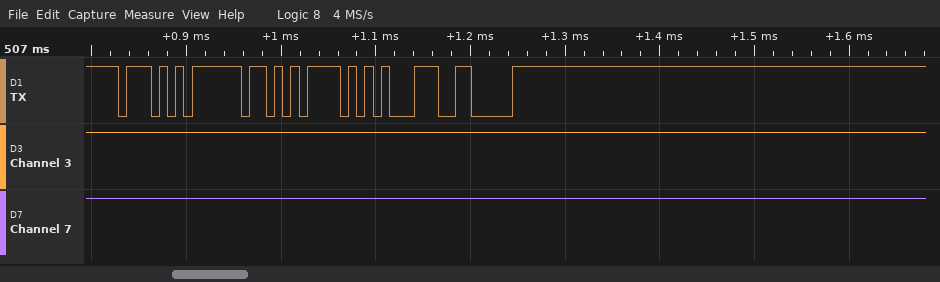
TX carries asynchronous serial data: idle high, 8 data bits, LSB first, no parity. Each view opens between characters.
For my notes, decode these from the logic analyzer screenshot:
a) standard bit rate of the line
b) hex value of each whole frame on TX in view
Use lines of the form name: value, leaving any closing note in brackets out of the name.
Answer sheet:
standard bit rate of the line: 115200 baud
hex value of each whole frame on TX in view: 57, AB, 15, 06
